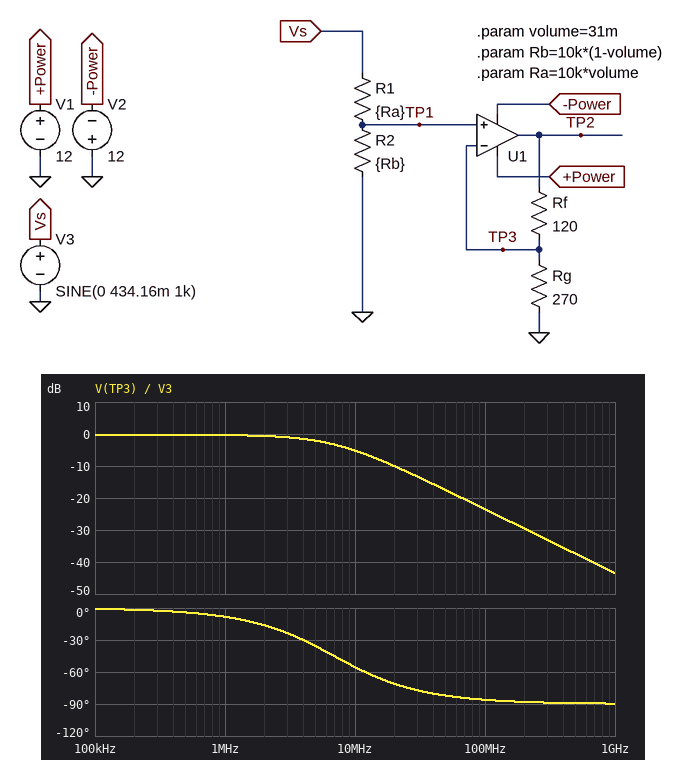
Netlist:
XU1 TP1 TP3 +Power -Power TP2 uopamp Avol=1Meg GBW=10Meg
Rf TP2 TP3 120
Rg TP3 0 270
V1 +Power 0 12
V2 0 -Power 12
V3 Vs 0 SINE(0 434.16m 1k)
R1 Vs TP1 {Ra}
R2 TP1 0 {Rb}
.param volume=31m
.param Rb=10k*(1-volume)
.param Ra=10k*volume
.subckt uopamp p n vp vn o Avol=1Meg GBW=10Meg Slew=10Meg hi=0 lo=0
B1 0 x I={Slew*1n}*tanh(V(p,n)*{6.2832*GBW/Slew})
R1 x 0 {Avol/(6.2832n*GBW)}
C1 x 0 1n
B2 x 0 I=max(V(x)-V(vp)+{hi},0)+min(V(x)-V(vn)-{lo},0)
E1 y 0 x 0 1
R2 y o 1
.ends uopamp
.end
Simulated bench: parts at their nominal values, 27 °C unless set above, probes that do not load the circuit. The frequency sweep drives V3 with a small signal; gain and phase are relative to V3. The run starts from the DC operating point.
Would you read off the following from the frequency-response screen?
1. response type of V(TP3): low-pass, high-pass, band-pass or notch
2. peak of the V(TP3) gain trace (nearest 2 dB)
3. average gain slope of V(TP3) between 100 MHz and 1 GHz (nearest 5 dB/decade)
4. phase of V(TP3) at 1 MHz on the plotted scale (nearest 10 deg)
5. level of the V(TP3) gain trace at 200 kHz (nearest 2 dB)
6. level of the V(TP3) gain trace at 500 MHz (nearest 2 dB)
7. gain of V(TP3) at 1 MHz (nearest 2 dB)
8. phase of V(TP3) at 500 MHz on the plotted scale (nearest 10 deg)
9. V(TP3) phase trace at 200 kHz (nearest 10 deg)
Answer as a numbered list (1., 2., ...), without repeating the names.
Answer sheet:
1. low-pass
2. 0 dB
3. -20 dB/decade
4. -10 deg
5. 0 dB
6. -38 dB
7. 0 dB
8. -90 deg
9. 0 deg
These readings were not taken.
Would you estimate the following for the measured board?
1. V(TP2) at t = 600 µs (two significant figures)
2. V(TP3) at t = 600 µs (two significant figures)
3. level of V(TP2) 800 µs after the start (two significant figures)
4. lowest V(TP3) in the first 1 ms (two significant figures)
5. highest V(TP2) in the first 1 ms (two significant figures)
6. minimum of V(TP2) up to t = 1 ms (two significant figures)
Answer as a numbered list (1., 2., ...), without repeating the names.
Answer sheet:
1. -360 mV
2. -250 mV
3. -580 mV
4. -420 mV
5. 610 mV
6. -610 mV
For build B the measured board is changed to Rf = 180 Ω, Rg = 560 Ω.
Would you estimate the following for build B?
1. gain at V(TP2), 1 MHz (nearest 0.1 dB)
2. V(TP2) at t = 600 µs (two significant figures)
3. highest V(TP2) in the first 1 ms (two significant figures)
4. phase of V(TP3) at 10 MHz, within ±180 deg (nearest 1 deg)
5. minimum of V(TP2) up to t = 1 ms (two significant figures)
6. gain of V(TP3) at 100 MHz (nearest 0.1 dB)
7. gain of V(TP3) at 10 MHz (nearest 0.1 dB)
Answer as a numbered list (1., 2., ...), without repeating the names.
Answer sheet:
1. 2.1 dB
2. -330 mV
3. 560 mV
4. -53 deg
5. -560 mV
6. -22.7 dB
7. -4.7 dB
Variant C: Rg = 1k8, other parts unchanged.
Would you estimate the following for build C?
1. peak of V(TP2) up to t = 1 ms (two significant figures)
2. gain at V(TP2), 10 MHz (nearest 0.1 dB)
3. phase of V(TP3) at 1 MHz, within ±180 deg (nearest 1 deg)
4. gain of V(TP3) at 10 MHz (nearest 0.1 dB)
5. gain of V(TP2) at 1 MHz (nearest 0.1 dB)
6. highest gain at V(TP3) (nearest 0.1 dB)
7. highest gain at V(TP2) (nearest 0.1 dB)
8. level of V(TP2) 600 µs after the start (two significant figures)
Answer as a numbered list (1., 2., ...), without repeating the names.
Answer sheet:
1. 450 mV
2. -3.0 dB
3. -6 deg
4. -3.6 dB
5. 0.2 dB
6. -0.3 dB
7. 0.3 dB
8. -260 mV
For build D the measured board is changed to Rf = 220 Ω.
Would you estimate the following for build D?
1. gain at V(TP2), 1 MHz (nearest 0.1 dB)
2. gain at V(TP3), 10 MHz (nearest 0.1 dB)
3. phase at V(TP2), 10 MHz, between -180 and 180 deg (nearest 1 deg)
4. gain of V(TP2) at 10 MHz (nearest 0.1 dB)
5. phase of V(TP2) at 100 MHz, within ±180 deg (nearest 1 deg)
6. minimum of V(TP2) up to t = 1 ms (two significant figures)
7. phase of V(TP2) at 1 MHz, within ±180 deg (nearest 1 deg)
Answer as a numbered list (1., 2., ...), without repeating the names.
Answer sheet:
1. 4.8 dB
2. -6.6 dB
3. -61 deg
4. -1.4 dB
5. -87 deg
6. -760 mV
7. -10 deg
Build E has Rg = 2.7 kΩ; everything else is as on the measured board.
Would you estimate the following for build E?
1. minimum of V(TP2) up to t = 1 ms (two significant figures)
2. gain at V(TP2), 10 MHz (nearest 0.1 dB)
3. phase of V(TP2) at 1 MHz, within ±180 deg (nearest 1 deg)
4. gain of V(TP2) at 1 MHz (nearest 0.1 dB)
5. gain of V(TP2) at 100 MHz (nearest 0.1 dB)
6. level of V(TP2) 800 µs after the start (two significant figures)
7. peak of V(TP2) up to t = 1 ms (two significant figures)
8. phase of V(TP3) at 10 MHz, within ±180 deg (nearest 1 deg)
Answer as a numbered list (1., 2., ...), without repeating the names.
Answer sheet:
1. -440 mV
2. -3.1 dB
3. -6 deg
4. 0.1 dB
5. -20.3 dB
6. -420 mV
7. 440 mV
8. -46 deg
